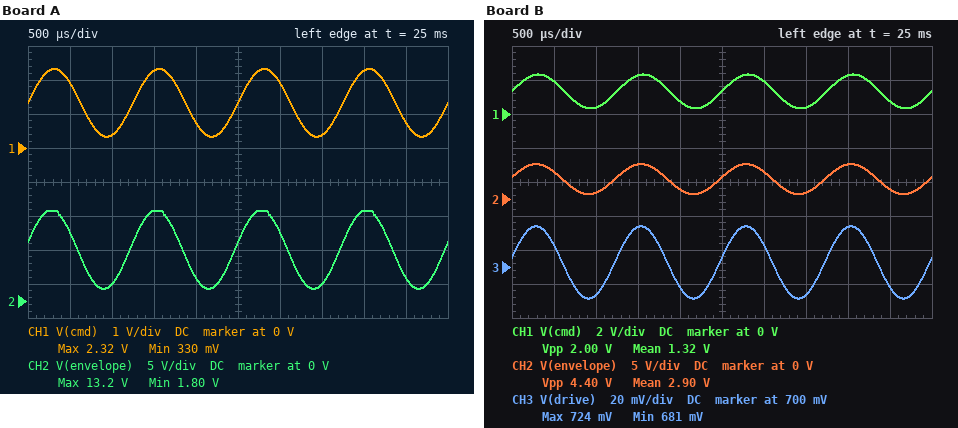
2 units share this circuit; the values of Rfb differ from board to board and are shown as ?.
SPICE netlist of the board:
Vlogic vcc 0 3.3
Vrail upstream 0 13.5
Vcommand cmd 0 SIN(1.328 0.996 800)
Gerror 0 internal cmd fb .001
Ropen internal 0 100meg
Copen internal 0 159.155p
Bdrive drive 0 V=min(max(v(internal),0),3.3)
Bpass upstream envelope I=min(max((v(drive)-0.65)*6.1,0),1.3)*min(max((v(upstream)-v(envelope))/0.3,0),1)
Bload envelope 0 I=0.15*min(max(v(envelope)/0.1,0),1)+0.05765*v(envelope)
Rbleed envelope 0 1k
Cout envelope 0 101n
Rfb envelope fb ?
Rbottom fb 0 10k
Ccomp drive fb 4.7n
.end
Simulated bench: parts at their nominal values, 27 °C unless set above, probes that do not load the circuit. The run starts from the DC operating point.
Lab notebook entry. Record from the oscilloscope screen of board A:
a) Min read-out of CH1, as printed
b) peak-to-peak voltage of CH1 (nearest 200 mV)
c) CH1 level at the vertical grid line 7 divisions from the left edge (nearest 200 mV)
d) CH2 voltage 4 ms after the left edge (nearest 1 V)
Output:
330 mV
2.0 V
400 mV
13 V
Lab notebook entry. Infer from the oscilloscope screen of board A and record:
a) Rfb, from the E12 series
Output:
47 kΩ
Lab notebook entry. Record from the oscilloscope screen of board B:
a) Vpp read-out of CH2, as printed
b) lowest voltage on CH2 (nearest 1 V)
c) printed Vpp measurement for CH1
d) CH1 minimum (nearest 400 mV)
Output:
4.40 V
1 V
2.00 V
400 mV
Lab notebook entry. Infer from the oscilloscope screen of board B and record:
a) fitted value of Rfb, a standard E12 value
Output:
12 kΩ
